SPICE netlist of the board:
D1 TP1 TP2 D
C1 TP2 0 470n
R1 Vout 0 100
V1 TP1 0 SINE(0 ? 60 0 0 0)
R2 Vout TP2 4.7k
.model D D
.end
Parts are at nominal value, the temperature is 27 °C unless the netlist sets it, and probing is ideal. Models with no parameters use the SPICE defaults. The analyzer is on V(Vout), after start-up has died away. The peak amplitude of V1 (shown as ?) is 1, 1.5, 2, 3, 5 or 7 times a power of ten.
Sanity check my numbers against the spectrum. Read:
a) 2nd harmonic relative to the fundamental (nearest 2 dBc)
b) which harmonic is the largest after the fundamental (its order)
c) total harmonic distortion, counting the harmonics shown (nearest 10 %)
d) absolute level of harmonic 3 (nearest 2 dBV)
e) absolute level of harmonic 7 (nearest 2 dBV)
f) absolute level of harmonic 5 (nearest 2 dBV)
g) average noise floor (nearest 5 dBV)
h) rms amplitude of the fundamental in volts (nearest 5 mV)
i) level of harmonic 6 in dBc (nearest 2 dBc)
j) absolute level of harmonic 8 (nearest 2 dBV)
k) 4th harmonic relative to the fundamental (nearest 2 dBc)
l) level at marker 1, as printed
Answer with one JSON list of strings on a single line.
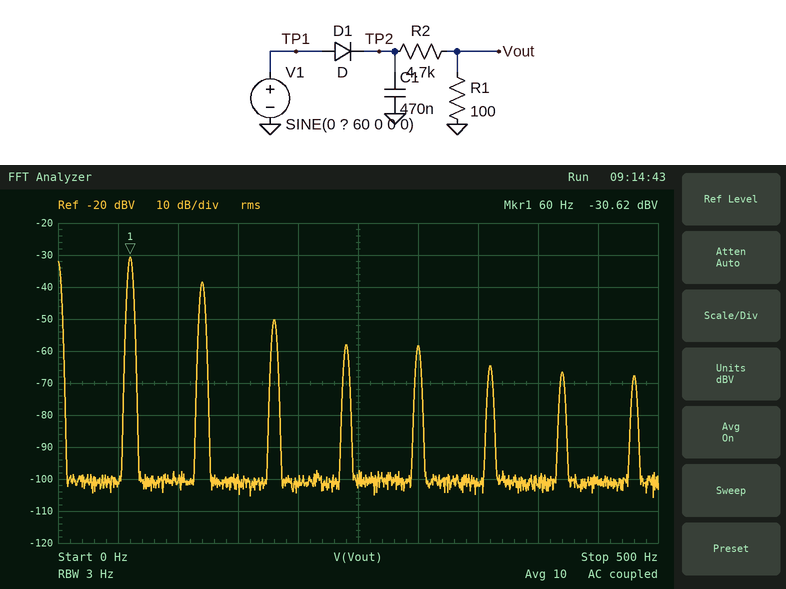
["-8 dBc", "2", "40 %", "-50 dBV", "-66 dBV", "-58 dBV", "-100 dBV", "30 mV", "-34 dBc", "-68 dBV", "-28 dBc", "-30.62 dBV"]
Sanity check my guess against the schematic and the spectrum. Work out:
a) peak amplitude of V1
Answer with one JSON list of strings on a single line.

["5 V"]
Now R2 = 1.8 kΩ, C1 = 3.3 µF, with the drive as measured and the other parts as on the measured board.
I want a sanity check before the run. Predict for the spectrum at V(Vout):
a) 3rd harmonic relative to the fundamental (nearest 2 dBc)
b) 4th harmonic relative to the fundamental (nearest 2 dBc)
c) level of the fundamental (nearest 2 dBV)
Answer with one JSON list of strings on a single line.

["-16 dBc", "-24 dBc", "-24 dBV"]
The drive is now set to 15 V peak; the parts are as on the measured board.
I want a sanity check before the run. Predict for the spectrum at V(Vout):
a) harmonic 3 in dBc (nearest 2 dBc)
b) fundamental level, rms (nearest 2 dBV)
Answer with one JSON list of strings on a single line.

["-22 dBc", "-20 dBV"]
